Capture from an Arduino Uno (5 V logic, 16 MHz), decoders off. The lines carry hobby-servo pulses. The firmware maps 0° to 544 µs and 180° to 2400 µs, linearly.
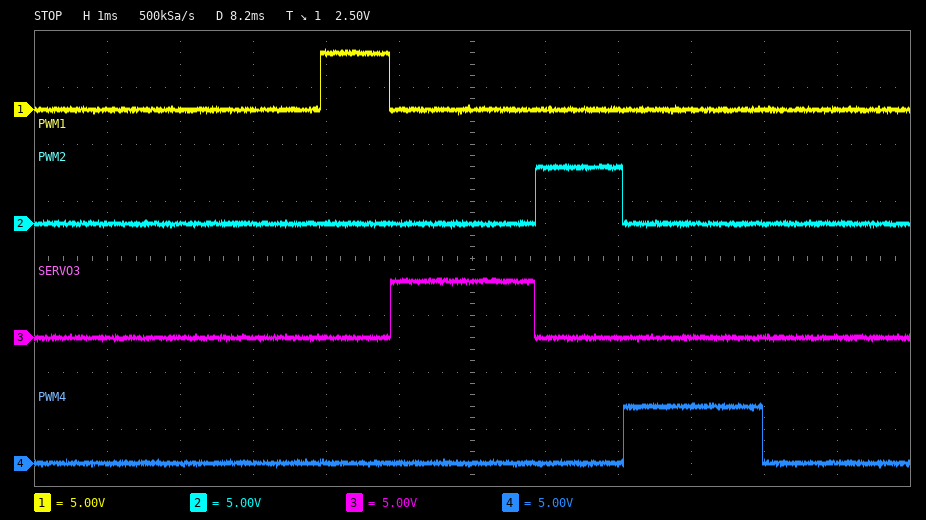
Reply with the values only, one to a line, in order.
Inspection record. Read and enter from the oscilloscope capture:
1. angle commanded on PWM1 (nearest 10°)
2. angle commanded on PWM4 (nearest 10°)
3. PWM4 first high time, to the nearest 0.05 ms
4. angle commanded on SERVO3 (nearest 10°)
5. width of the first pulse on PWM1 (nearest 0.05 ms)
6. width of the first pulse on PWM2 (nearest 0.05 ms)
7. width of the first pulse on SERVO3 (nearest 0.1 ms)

40°
130°
1.90 ms
140°
0.95 ms
1.20 ms
2.0 ms
